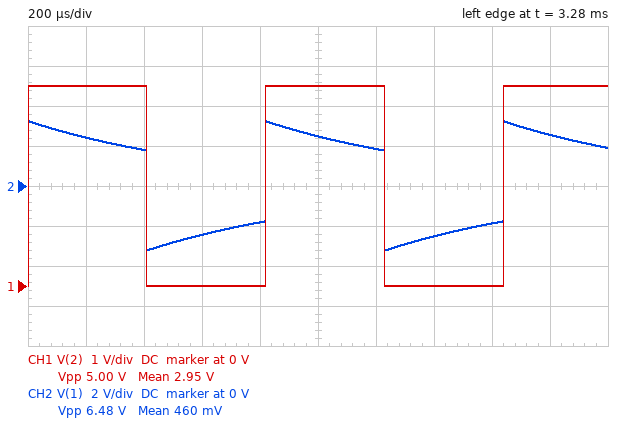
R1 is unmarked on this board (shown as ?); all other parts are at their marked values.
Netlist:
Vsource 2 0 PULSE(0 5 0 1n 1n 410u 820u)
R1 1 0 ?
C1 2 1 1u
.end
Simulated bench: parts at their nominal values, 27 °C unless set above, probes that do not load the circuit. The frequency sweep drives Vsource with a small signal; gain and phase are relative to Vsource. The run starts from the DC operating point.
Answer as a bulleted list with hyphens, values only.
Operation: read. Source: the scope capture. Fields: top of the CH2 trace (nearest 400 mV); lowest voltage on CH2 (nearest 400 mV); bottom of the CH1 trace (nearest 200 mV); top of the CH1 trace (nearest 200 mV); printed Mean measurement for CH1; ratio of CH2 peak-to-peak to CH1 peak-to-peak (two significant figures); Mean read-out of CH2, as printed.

- 3.2 V
- -3.2 V
- 0 V
- 5.0 V
- 2.95 V
- 1.3
- 460 mV
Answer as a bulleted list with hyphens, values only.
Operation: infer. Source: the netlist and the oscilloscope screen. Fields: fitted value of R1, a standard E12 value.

- 680 Ω
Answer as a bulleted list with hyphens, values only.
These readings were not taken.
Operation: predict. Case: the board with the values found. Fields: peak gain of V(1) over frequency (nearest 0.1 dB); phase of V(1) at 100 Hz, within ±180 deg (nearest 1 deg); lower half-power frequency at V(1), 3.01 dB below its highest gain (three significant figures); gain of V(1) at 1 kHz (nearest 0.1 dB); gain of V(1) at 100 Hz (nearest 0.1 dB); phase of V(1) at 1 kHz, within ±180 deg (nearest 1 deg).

- 0 dB
- 67 deg
- 234 Hz
- -0.2 dB
- -8.1 dB
- 13 deg
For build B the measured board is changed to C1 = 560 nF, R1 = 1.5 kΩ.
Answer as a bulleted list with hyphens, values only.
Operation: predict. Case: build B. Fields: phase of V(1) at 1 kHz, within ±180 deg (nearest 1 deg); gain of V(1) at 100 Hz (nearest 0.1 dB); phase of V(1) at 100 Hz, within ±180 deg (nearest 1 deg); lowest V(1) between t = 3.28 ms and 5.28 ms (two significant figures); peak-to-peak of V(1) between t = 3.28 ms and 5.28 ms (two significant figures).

- 11 deg
- -6.6 dB
- 62 deg
- -3.1 V
- 6.2 V
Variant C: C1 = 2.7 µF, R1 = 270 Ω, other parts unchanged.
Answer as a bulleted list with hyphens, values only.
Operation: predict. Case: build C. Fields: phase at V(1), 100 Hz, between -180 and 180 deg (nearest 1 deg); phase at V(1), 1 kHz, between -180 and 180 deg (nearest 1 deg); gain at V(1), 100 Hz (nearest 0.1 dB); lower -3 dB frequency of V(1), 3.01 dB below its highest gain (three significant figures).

- 65 deg
- 12 deg
- -7.6 dB
- 218 Hz
